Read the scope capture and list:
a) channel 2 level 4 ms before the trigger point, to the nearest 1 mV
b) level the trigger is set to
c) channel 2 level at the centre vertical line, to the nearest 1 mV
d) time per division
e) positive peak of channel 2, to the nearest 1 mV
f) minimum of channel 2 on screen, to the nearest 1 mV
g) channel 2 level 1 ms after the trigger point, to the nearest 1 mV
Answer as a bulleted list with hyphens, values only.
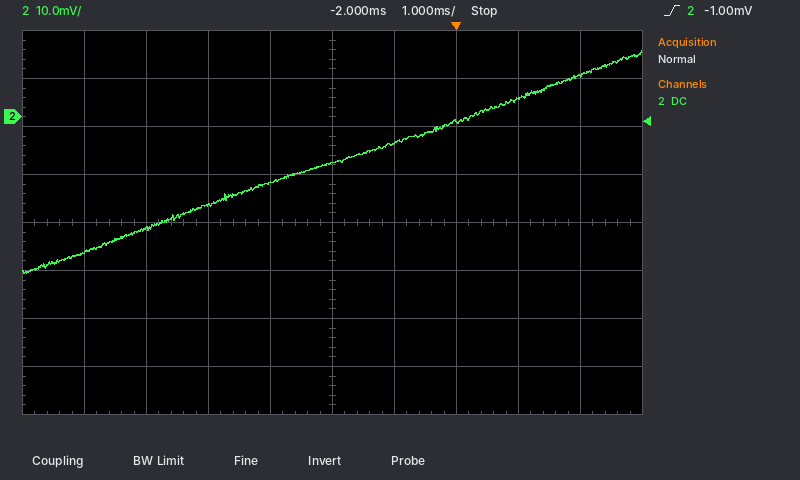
- -18 mV
- -1.00 mV
- -10 mV
- 1 ms
- 14 mV
- -33 mV
- 4 mV
